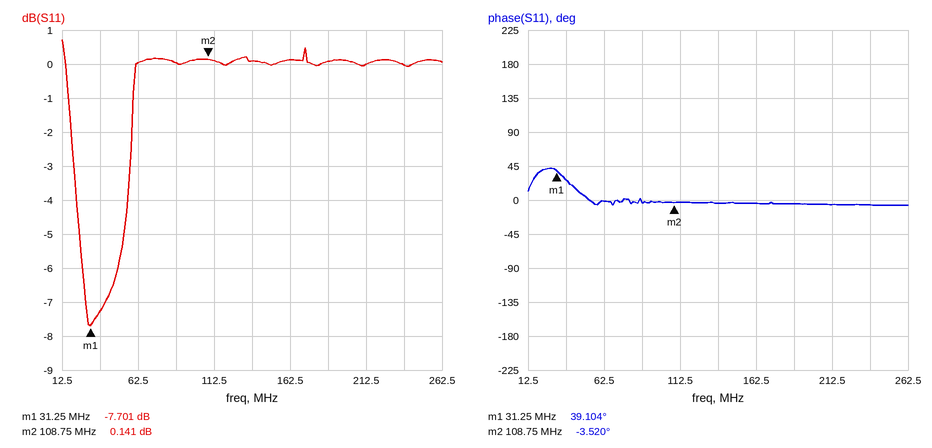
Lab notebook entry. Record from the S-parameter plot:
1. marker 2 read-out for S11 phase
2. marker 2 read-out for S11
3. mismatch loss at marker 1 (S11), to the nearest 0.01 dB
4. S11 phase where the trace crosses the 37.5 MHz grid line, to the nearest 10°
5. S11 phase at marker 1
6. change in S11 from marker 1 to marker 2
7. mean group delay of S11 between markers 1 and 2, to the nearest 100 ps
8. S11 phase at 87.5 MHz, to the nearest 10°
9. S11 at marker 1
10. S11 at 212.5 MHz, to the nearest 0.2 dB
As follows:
-3.520°
0.141 dB
0.81 dB
30°
39.104°
7.842 dB
1.5 ns
0°
-7.701 dB
0.0 dB
